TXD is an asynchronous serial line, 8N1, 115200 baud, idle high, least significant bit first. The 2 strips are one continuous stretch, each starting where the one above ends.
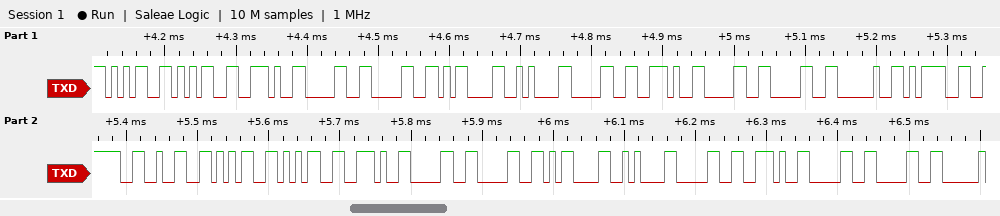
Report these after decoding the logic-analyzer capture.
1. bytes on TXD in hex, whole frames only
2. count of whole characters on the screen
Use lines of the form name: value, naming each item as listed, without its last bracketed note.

bytes on TXD in hex, whole frames only: 35 35 2E 30 30 0D 0A 30 2E 30 30 20 3D 3E 32 35 35 2E 30 30 0D 0A 30 2E 30 30
count of whole characters on the screen: 26
